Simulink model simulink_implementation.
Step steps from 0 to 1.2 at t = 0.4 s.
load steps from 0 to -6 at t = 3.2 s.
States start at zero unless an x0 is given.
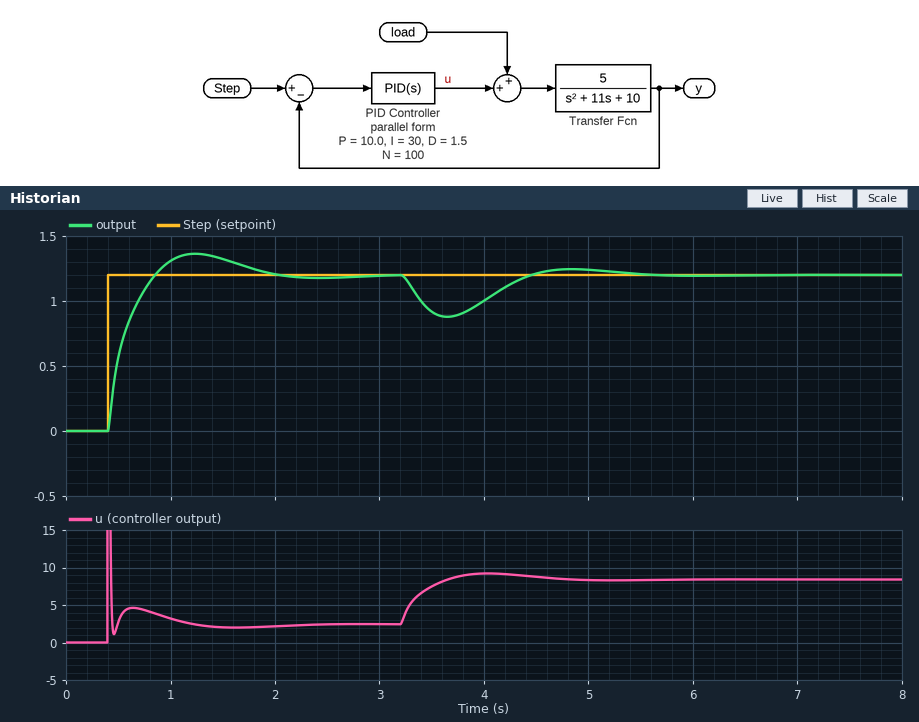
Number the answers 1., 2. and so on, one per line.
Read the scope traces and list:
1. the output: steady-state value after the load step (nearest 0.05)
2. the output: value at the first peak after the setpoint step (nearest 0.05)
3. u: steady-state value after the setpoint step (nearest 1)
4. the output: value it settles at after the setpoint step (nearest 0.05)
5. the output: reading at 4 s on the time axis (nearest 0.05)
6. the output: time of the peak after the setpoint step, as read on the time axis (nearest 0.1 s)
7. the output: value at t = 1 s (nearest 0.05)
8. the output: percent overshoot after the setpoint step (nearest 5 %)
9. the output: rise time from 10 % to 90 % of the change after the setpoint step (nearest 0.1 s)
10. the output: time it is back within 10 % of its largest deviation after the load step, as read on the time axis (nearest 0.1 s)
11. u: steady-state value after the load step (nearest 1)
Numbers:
1. 1.20
2. 1.35
3. 2
4. 1.20
5. 1.00
6. 1.2 s
7. 1.30
8. 15 %
9. 0.3 s
10. 5.1 s
11. 8
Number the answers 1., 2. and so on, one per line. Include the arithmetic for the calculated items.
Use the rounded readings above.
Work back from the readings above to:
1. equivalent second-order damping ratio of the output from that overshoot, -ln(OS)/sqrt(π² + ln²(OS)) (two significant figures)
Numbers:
1. ln(0.15) = -1.897; 1.897 / sqrt(9.870 + 3.599) = 0.52
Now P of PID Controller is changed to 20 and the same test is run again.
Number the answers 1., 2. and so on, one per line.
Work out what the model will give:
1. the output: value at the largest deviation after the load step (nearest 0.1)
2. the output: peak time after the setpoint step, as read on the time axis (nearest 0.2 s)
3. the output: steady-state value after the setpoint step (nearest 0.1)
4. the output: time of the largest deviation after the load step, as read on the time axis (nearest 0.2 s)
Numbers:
1. 1.0
2. 1.0 s
3. 1.2
4. 3.6 s
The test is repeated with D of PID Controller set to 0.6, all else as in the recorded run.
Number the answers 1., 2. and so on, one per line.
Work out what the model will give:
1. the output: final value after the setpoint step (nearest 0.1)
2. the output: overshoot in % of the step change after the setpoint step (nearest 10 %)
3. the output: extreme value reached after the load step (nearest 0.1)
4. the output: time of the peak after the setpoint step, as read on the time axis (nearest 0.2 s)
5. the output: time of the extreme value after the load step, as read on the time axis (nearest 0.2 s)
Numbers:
1. 1.2
2. 20 %
3. 0.8
4. 1.0 s
5. 3.6 s
